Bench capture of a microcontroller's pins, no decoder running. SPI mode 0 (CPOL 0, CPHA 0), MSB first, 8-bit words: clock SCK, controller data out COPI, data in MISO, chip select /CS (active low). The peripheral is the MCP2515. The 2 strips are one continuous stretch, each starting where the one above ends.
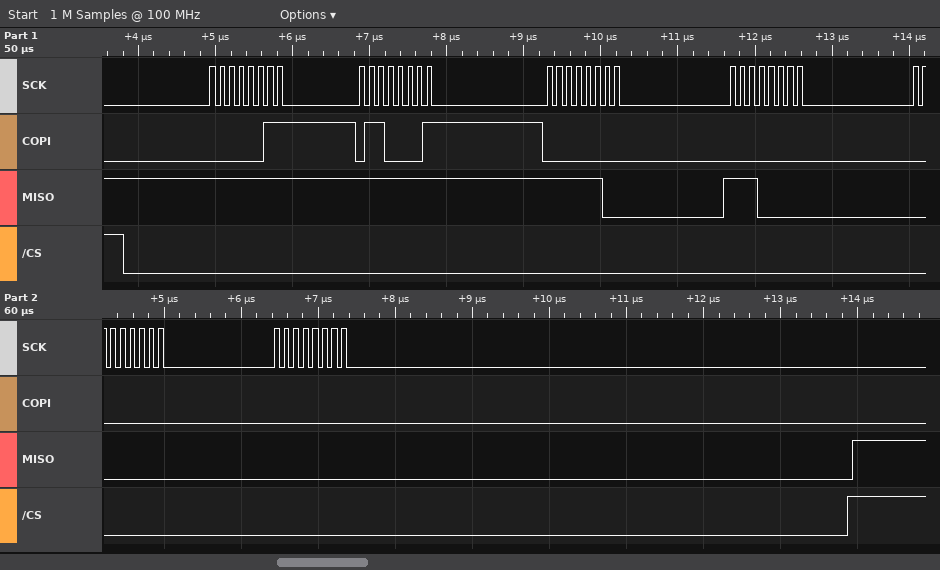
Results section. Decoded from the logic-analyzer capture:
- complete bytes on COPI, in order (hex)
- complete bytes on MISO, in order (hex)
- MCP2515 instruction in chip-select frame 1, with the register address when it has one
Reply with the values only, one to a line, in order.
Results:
0x03 0x61 0x00 0x00 0x00 0x00
0xFF 0xFF 0xFC 0xE0 0x00 0x00
READ 0x61
